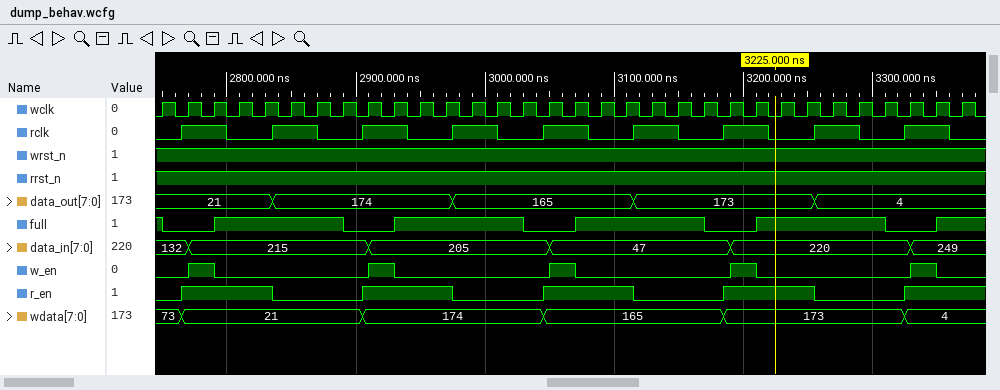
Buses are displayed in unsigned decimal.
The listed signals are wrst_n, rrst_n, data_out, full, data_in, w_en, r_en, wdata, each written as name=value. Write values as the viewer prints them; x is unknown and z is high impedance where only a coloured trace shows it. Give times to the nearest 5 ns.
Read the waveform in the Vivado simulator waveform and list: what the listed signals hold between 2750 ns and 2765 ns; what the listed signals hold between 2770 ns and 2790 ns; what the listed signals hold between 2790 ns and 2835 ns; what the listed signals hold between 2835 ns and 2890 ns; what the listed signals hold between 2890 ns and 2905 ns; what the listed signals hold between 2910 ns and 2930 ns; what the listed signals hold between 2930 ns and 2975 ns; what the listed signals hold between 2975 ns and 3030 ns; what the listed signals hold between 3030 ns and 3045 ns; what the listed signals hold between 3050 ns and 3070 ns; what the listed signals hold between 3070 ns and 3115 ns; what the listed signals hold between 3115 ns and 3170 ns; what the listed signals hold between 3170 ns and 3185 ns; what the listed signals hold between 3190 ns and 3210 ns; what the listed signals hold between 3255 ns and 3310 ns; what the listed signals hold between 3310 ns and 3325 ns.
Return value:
wrst_n=1, rrst_n=1, data_out=21, full=0, data_in=132, w_en=0, r_en=0, wdata=73
wrst_n=1, rrst_n=1, data_out=21, full=0, data_in=215, w_en=1, r_en=1, wdata=21
wrst_n=1, rrst_n=1, data_out=21, full=1, data_in=215, w_en=0, r_en=1, wdata=21
wrst_n=1, rrst_n=1, data_out=174, full=1, data_in=215, w_en=0, r_en=0, wdata=21
wrst_n=1, rrst_n=1, data_out=174, full=0, data_in=215, w_en=0, r_en=0, wdata=21
wrst_n=1, rrst_n=1, data_out=174, full=0, data_in=205, w_en=1, r_en=1, wdata=174
wrst_n=1, rrst_n=1, data_out=174, full=1, data_in=205, w_en=0, r_en=1, wdata=174
wrst_n=1, rrst_n=1, data_out=165, full=1, data_in=205, w_en=0, r_en=0, wdata=174
wrst_n=1, rrst_n=1, data_out=165, full=0, data_in=205, w_en=0, r_en=0, wdata=174
wrst_n=1, rrst_n=1, data_out=165, full=0, data_in=47, w_en=1, r_en=1, wdata=165
wrst_n=1, rrst_n=1, data_out=165, full=1, data_in=47, w_en=0, r_en=1, wdata=165
wrst_n=1, rrst_n=1, data_out=173, full=1, data_in=47, w_en=0, r_en=0, wdata=165
wrst_n=1, rrst_n=1, data_out=173, full=0, data_in=47, w_en=0, r_en=0, wdata=165
wrst_n=1, rrst_n=1, data_out=173, full=0, data_in=220, w_en=1, r_en=1, wdata=173
wrst_n=1, rrst_n=1, data_out=4, full=1, data_in=220, w_en=0, r_en=0, wdata=173
wrst_n=1, rrst_n=1, data_out=4, full=0, data_in=220, w_en=0, r_en=0, wdata=173
